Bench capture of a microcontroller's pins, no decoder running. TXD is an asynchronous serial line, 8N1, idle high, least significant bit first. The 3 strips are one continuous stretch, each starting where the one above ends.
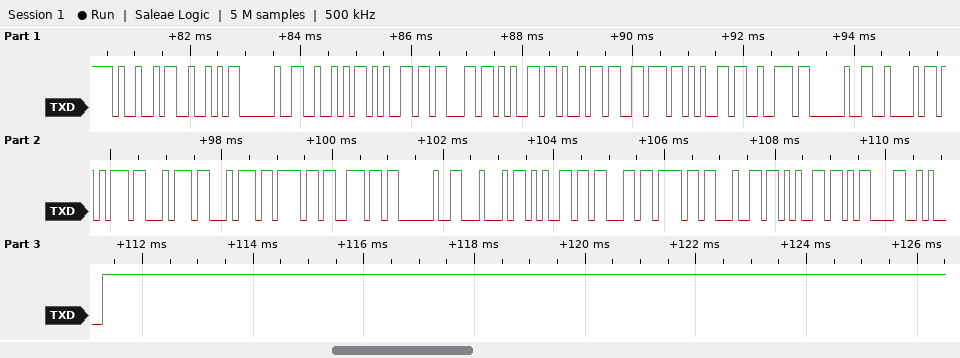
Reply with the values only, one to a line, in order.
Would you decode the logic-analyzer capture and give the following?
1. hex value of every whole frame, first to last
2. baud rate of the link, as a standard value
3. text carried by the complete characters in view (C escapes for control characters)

0x49 0x52 0x20 0x52 0x65 0x63 0x65 0x69 0x76 0x65 0x72 0x20 0x42 0x75 0x74 0x74 0x6F 0x6E 0x20 0x44 0x65 0x63 0x6F 0x64 0x65 0x0D 0x0A
9600 baud
"IR Receiver Button Decode\r\n"
